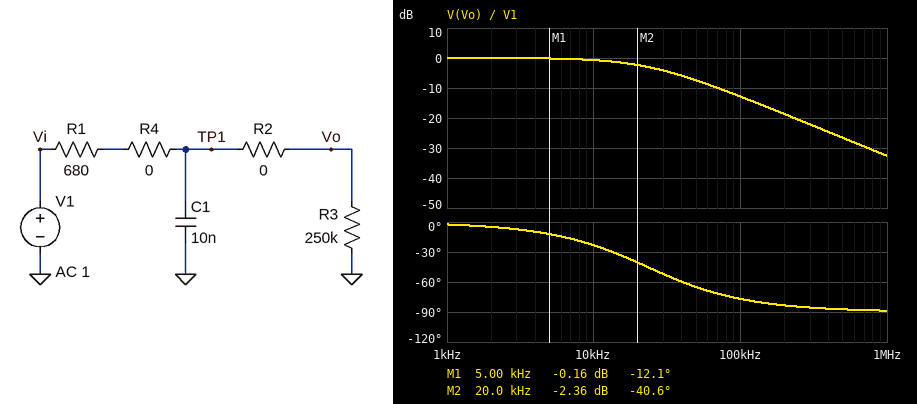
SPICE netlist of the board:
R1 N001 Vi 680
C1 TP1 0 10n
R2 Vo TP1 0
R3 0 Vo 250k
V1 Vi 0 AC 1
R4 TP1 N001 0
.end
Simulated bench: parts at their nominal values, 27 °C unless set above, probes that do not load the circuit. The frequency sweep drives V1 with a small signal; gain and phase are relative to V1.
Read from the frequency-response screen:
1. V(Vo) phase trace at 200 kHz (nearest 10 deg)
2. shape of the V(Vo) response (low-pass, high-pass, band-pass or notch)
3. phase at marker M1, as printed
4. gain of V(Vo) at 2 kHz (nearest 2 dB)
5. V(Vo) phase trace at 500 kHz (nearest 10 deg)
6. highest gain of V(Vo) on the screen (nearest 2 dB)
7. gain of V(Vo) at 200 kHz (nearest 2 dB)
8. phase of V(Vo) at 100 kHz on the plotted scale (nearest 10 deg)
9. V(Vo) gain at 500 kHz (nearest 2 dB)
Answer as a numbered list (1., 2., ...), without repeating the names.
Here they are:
1. -80 deg
2. low-pass
3. -12.1 deg
4. 0 dB
5. -90 deg
6. 0 dB
7. -18 dB
8. -80 deg
9. -26 dB
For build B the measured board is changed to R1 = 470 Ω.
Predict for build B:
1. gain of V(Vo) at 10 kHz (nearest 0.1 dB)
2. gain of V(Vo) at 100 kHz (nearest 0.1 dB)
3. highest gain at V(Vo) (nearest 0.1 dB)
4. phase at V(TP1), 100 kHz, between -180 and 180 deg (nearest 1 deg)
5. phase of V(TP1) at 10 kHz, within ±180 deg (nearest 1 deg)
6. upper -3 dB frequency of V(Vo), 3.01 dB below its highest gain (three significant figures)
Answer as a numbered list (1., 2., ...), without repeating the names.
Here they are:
1. 0.3 dB
2. -9.8 dB
3. 0.7 dB
4. -73 deg
5. -18 deg
6. 31.1 kHz
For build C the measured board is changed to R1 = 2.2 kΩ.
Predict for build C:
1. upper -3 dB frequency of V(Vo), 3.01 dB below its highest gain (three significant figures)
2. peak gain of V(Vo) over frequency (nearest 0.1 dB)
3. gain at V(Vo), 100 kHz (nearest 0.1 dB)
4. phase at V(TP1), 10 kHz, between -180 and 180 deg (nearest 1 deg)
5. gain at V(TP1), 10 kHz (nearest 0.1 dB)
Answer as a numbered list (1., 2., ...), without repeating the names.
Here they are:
1. 7.77 kHz
2. -0.6 dB
3. -22.8 dB
4. -52 deg
5. -4.9 dB
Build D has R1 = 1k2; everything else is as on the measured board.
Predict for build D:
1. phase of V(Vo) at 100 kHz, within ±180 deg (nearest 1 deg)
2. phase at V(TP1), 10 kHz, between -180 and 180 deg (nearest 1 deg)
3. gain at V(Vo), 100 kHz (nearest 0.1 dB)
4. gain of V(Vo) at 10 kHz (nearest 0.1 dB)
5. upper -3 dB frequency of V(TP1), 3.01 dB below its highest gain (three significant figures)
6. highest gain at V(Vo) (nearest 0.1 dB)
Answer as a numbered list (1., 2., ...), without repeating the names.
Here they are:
1. -83 deg
2. -41 deg
3. -17.6 dB
4. -1.3 dB
5. 11.7 kHz
6. 1.1 dB
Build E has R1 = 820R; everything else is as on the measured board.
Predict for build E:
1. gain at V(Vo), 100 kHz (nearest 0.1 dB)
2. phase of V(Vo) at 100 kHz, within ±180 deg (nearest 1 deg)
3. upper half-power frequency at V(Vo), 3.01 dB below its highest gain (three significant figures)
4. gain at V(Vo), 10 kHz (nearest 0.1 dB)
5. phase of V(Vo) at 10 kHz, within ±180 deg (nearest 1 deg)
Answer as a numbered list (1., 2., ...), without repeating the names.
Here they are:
1. -14.4 dB
2. -79 deg
3. 19.4 kHz
4. -1.0 dB
5. -27 deg
